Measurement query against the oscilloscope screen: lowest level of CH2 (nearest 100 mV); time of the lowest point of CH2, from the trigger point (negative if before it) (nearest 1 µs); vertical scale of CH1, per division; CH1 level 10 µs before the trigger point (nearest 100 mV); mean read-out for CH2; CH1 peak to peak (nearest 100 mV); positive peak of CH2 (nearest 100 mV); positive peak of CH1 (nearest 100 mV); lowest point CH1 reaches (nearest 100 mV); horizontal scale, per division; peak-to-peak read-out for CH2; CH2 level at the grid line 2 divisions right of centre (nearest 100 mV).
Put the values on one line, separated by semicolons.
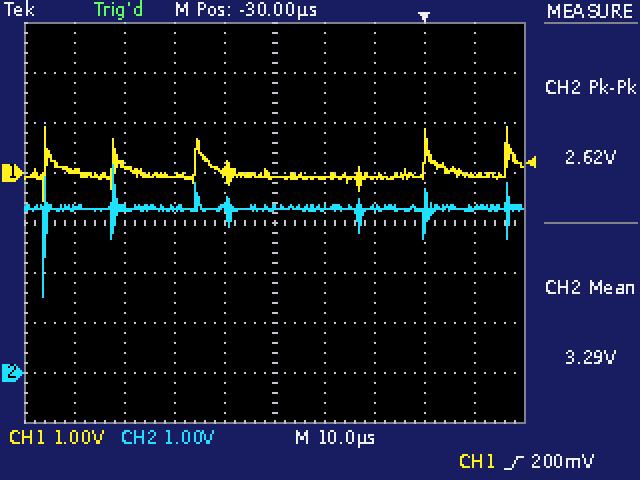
1.5 V; -76 µs; 1 V; -100 mV; 3.29 V; 1.5 V; 4.2 V; 900 mV; -600 mV; 10 µs; 2.62 V; 3.3 V
